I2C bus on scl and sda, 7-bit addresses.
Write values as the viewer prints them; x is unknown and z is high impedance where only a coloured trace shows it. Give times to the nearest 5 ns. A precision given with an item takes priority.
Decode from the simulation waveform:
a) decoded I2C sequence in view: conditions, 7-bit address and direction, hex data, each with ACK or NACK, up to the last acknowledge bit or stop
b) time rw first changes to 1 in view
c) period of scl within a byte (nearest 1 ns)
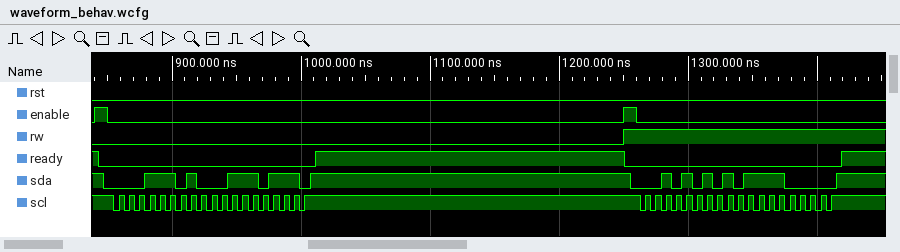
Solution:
start, address 0E read ACK, 3B NACK, stop, start, address 15 write NACK, 78 ACK, stop
1250 ns
8 ns
